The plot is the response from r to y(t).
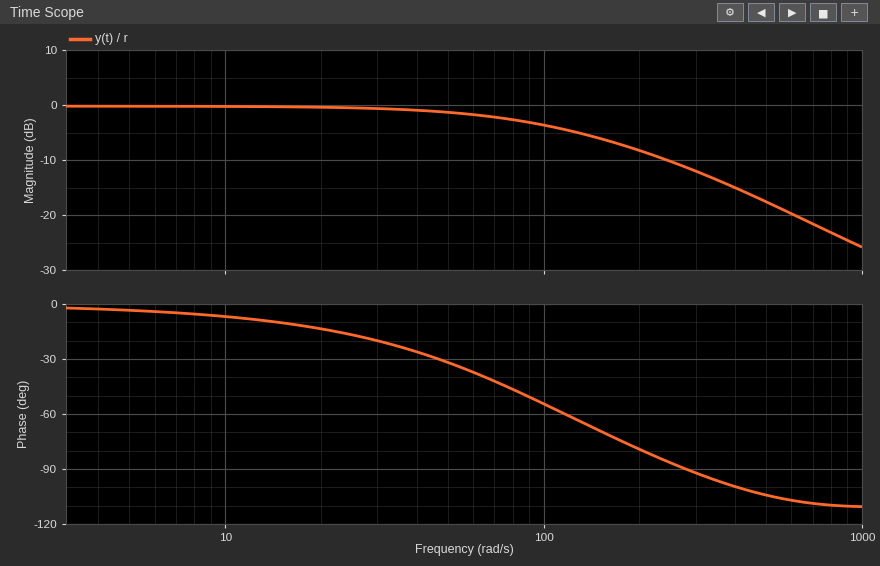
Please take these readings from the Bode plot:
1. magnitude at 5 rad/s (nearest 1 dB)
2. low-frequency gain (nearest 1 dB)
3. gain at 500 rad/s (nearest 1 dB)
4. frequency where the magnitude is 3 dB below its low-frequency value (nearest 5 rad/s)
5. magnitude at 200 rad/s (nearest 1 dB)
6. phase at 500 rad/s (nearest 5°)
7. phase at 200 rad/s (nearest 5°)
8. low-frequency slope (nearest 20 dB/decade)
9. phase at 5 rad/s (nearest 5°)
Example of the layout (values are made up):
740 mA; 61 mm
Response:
0 dB; 0 dB; -18 dB; 90 rad/s; -8 dB; -105°; -80°; 0 dB/decade; -5°
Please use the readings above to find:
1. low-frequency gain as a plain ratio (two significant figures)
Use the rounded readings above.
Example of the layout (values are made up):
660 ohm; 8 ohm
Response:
1.0
